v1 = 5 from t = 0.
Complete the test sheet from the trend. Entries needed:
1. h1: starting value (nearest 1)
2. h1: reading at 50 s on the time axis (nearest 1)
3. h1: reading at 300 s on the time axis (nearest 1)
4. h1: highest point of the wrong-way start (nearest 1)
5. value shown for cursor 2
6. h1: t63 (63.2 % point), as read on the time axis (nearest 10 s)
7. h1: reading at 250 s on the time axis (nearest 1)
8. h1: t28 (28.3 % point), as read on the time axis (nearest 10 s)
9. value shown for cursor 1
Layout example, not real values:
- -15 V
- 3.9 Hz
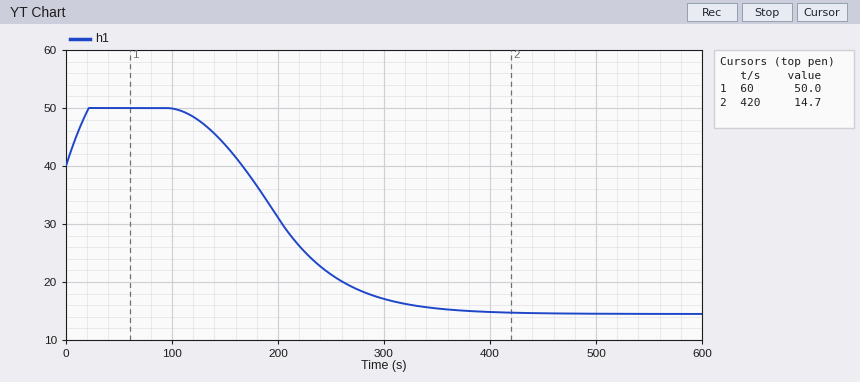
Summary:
- 40
- 50
- 17
- 50
- 14.7
- 230 s
- 21
- 190 s
- 50.0
